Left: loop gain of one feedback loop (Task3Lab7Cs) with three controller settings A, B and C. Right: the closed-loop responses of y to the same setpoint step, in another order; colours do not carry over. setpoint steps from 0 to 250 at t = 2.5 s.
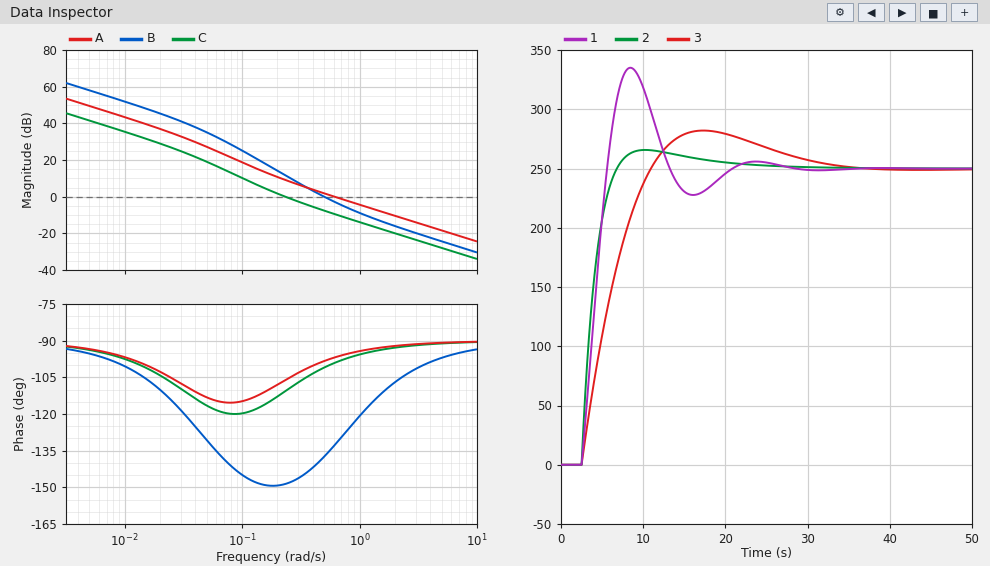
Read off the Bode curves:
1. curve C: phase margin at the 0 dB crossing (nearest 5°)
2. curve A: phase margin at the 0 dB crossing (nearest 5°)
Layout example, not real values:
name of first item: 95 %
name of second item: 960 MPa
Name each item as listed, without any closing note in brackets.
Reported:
curve C: phase margin at the 0 dB crossing: 70°
curve A: phase margin at the 0 dB crossing: 85°
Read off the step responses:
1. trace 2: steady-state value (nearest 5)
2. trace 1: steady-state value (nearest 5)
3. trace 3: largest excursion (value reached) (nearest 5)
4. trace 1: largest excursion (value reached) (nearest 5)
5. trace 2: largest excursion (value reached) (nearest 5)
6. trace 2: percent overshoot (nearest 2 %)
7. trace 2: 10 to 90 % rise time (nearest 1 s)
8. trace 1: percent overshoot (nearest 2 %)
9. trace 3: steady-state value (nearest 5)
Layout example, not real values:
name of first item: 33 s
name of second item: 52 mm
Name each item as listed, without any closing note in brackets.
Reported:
trace 2: steady-state value: 250
trace 1: steady-state value: 250
trace 3: largest excursion (value reached): 280
trace 1: largest excursion (value reached): 335
trace 2: largest excursion (value reached): 265
trace 2: percent overshoot: 6 %
trace 2: 10 to 90 % rise time: 3 s
trace 1: percent overshoot: 34 %
trace 3: steady-state value: 250
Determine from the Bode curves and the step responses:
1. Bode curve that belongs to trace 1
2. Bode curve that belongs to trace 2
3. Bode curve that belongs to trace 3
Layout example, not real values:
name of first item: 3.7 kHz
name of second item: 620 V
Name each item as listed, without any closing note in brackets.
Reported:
Bode curve that belongs to trace 1: B
Bode curve that belongs to trace 2: A
Bode curve that belongs to trace 3: C
